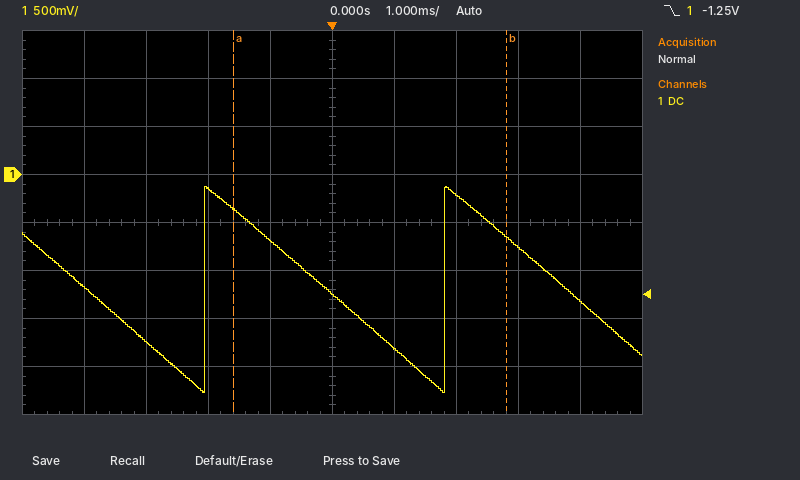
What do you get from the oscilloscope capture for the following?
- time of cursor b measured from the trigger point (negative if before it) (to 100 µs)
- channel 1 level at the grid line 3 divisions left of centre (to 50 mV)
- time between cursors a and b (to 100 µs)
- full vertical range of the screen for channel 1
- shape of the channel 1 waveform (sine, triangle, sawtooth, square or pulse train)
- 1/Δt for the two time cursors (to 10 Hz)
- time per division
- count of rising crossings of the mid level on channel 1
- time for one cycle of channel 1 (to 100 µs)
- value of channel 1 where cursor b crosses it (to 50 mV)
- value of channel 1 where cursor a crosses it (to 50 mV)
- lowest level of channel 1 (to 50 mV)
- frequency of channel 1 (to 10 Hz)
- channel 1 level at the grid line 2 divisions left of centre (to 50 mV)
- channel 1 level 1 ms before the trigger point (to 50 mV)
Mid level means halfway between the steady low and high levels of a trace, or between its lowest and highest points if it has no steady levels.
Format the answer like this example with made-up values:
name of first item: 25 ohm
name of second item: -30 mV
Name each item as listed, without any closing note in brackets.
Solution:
time of cursor b measured from the trigger point (negative if before it): +2.8 ms
channel 1 level at the grid line 3 divisions left of centre: -1.75 V
time between cursors a and b: 4.4 ms
full vertical range of the screen for channel 1: 4 V
shape of the channel 1 waveform: sawtooth
1/Δt for the two time cursors: 230 Hz
time per division: 1 ms
count of rising crossings of the mid level on channel 1: 2
time for one cycle of channel 1: 3.9 ms
value of channel 1 where cursor b crosses it: -650 mV
value of channel 1 where cursor a crosses it: -350 mV
lowest level of channel 1: -2.25 V
frequency of channel 1: 260 Hz
channel 1 level at the grid line 2 divisions left of centre: -150 mV
channel 1 level 1 ms before the trigger point: -700 mV
